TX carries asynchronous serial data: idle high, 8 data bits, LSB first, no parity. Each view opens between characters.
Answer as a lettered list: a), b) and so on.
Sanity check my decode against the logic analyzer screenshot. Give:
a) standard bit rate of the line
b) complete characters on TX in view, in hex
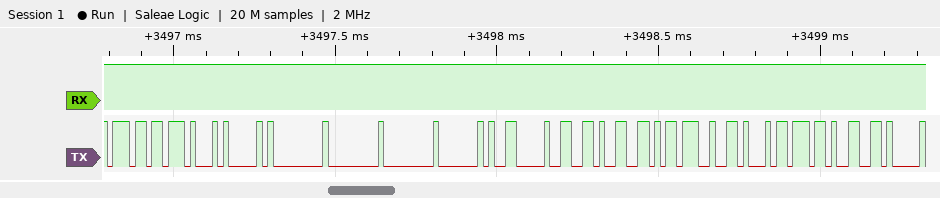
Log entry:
a) 57600 baud
b) B7, 17, 41, 00, 00, 00, 40, 06, 66, 66, 3B, 16, BB, 99
